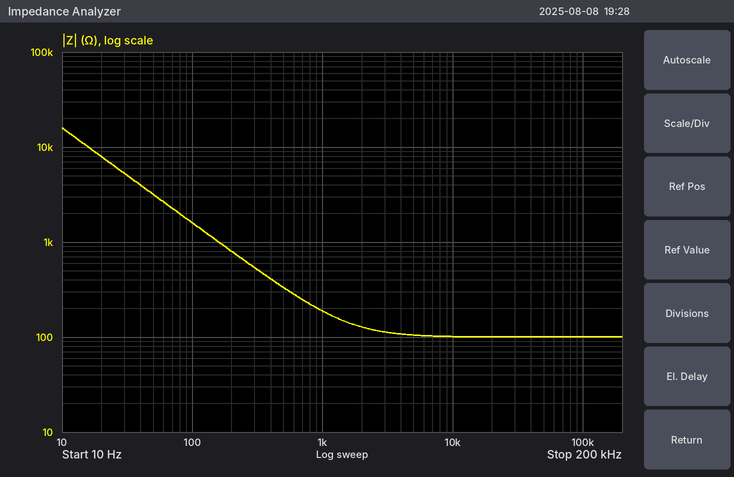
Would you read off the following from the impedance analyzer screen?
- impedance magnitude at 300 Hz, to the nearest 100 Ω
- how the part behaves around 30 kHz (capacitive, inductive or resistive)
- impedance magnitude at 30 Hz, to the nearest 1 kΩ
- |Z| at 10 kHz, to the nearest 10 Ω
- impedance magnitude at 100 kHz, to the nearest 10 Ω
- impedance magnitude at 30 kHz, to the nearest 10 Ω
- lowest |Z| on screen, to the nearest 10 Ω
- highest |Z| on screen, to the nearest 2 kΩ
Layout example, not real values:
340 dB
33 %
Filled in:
500 Ω
resistive
5 kΩ
100 Ω
100 Ω
100 Ω
100 Ω
16 kΩ
